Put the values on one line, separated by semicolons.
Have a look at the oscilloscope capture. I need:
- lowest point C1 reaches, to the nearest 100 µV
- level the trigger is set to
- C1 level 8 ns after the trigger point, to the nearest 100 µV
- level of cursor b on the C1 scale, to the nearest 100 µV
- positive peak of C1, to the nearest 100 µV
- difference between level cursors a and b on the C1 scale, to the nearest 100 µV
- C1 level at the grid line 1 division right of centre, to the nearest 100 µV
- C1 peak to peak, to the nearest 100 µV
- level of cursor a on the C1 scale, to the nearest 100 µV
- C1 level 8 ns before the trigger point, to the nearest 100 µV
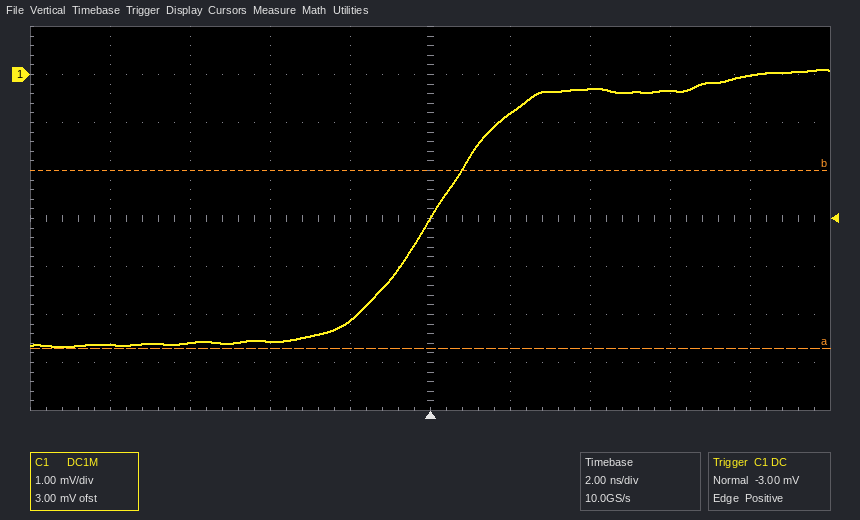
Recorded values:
-5.7 mV; -3.00 mV; 0.0 mV; -2.0 mV; 100 µV; 3.7 mV; -800 µV; 5.8 mV; -5.7 mV; -5.6 mV
